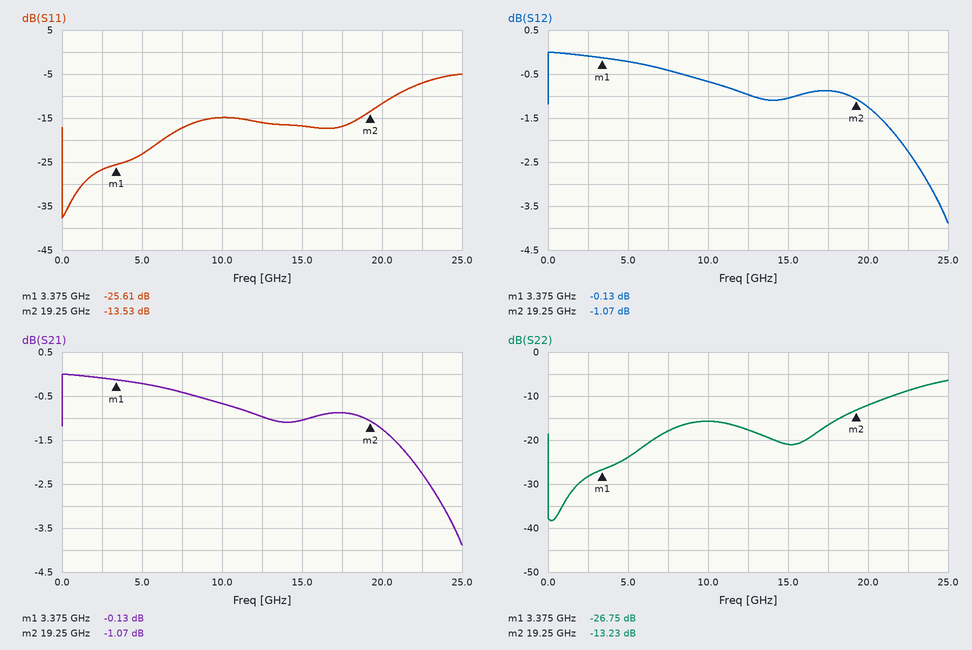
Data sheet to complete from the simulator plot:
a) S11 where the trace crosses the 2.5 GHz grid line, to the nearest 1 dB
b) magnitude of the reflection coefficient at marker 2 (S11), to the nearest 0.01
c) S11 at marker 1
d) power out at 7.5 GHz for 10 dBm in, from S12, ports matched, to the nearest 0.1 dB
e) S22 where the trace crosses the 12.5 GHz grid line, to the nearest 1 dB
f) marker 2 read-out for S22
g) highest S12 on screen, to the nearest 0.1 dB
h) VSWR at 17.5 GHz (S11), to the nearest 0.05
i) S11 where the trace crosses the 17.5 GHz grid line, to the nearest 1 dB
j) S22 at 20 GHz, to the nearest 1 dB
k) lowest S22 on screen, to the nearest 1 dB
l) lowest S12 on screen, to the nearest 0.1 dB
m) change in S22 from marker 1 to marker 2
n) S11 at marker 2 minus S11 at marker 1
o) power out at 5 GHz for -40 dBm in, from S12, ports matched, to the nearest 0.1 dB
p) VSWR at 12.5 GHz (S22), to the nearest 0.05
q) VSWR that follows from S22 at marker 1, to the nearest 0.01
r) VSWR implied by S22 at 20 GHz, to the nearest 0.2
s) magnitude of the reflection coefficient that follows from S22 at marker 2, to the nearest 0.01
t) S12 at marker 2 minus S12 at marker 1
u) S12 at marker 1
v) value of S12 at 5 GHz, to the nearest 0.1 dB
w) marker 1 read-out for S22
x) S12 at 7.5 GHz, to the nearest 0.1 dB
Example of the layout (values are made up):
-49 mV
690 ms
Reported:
-27 dB
0.21
-25.61 dB
9.6 dBm
-18 dB
-13.23 dB
0.0 dB
1.35
-17 dB
-12 dB
-38 dB
-3.9 dB
13.52 dB
12.08 dB
-40.2 dBm
1.30
1.10
1.6
0.22
-0.94 dB
-0.13 dB
-0.2 dB
-26.75 dB
-0.4 dB
